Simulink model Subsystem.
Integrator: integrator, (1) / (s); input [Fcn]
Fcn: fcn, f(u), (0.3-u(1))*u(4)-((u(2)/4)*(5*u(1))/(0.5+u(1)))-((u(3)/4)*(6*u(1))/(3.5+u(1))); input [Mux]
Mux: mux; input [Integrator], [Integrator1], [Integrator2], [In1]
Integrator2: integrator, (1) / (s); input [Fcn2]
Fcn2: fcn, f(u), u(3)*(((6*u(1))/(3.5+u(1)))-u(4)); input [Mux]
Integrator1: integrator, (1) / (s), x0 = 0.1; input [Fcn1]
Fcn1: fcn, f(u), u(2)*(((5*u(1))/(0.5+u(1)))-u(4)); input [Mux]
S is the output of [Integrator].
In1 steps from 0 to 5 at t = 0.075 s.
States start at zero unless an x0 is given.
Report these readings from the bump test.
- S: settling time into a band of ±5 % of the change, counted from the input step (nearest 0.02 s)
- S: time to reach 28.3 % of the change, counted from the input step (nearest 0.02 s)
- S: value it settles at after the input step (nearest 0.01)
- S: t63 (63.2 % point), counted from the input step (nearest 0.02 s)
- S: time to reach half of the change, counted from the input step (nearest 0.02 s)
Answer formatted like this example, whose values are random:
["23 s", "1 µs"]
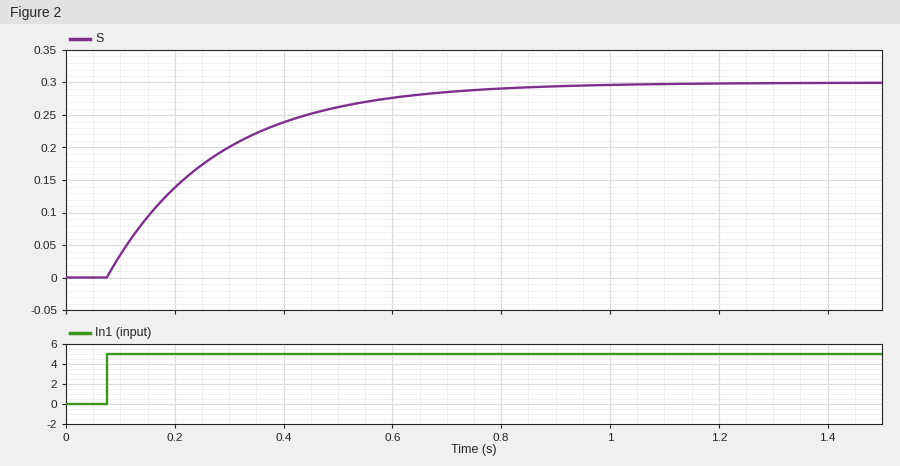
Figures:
["0.62 s", "0.06 s", "0.30", "0.20 s", "0.14 s"]
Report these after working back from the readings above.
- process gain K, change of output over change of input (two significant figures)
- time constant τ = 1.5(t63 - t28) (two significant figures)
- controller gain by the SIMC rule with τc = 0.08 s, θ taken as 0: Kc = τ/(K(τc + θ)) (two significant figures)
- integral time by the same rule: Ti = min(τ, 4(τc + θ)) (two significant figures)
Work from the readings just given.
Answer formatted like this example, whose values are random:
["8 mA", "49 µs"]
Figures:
["0.060", "0.21 s", "44", "0.21 s"]
